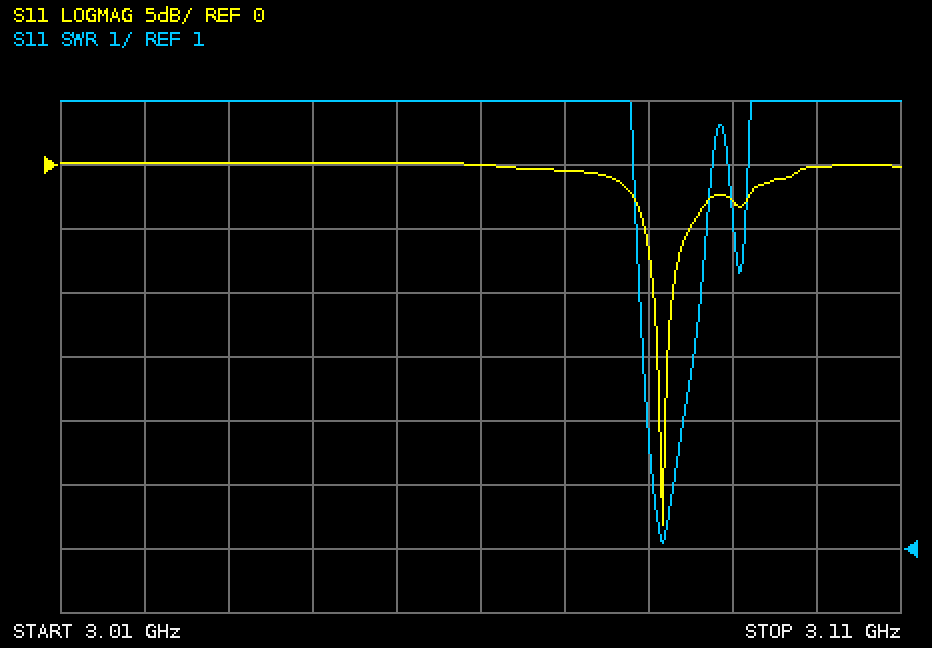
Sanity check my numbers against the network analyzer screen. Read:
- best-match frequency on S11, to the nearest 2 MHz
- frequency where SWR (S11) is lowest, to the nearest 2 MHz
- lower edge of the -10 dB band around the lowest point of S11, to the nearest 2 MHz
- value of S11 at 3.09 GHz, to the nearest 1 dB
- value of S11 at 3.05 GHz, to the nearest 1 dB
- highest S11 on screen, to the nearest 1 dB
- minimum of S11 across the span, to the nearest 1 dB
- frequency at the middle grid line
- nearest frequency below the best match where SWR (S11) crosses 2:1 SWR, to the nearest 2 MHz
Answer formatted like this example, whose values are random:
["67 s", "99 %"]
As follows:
["3.082 GHz", "3.082 GHz", "3.080 GHz", "-3 dB", "0 dB", "0 dB", "-28 dB", "3.06 GHz", "3.080 GHz"]
